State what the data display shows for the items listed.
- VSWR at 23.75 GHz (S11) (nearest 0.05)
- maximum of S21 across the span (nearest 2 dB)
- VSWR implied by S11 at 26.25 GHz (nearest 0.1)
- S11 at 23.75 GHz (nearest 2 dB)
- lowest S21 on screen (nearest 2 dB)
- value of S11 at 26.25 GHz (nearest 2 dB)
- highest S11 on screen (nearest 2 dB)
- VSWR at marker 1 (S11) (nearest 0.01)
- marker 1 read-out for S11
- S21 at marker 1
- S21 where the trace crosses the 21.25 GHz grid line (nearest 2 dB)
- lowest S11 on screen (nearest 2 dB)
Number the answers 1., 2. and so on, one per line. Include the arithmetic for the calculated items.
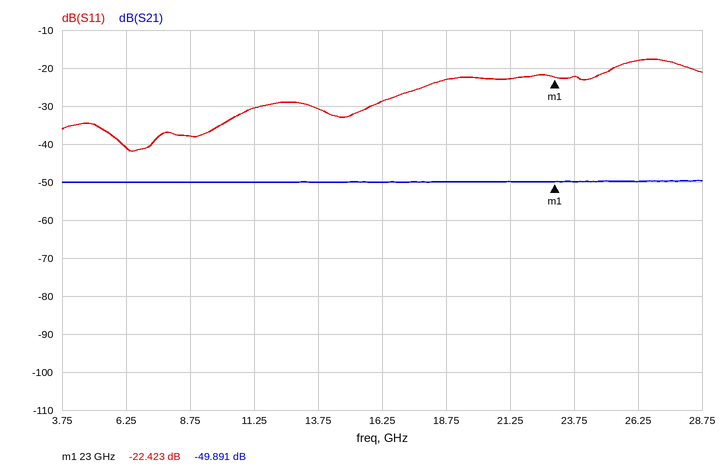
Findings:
1. |Γ| = 10^(-22/20) = 0.0794; VSWR = (1 + 0.0794)/(1 − 0.0794) ≈ 1.17, so 1.15 to the nearest 0.05
2. -50 dB
3. |Γ| = 10^(-18/20) = 0.1259; VSWR = (1 + 0.1259)/(1 − 0.1259) ≈ 1.3
4. -22 dB
5. -50 dB
6. -18 dB
7. -18 dB
8. (1 + 0.0757)/(1 − 0.0757) ≈ 1.16
9. -22.423 dB
10. -49.891 dB
11. -50 dB
12. -42 dB
